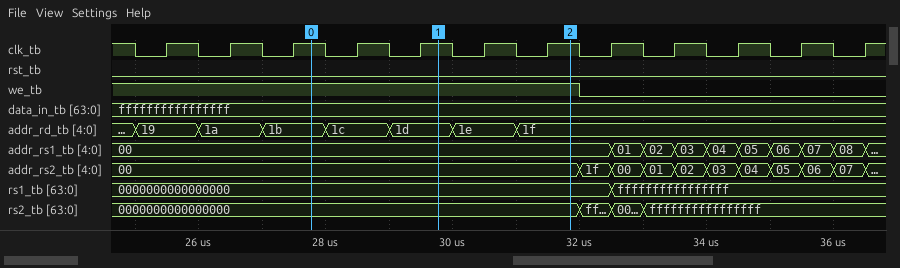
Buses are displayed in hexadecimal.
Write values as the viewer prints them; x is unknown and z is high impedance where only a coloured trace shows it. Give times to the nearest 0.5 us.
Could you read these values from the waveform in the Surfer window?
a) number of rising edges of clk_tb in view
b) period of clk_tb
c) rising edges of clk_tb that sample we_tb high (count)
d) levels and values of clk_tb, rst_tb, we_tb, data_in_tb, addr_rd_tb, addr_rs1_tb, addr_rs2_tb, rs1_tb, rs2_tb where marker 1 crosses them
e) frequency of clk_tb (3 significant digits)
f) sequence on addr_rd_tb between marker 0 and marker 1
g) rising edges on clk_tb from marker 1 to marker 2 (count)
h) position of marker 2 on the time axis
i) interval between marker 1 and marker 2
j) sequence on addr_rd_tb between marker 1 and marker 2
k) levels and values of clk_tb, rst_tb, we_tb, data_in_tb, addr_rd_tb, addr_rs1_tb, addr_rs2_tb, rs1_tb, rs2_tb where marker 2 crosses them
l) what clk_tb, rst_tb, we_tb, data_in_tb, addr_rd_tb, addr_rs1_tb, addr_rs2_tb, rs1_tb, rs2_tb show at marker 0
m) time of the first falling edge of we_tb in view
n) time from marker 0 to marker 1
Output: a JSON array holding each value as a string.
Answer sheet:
["12", "1 us", "7", "clk_tb=1, rst_tb=0, we_tb=1, data_in_tb=ffffffffffffffff, addr_rd_tb=1d, addr_rs1_tb=00, addr_rs2_tb=00, rs1_tb=0000000000000000, rs2_tb=0000000000000000", "1.00 MHz", "1b, 1c, 1d", "2", "32 us", "2 us", "1d, 1e, 1f", "clk_tb=1, rst_tb=0, we_tb=1, data_in_tb=ffffffffffffffff, addr_rd_tb=1f, addr_rs1_tb=00, addr_rs2_tb=00, rs1_tb=0000000000000000, rs2_tb=0000000000000000", "clk_tb=1, rst_tb=0, we_tb=1, data_in_tb=ffffffffffffffff, addr_rd_tb=1b, addr_rs1_tb=00, addr_rs2_tb=00, rs1_tb=0000000000000000, rs2_tb=0000000000000000", "32 us", "2 us"]
